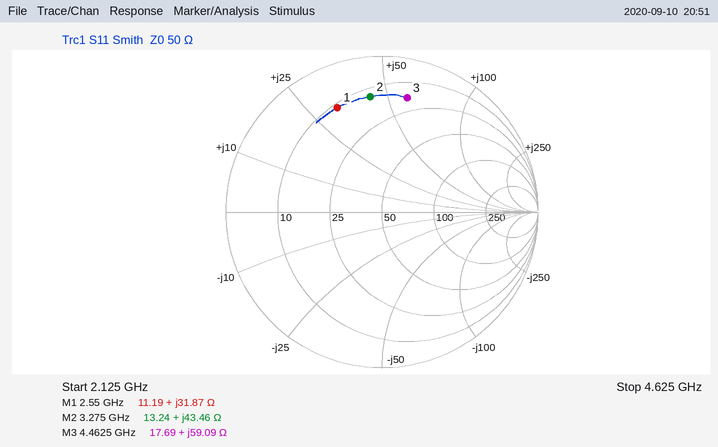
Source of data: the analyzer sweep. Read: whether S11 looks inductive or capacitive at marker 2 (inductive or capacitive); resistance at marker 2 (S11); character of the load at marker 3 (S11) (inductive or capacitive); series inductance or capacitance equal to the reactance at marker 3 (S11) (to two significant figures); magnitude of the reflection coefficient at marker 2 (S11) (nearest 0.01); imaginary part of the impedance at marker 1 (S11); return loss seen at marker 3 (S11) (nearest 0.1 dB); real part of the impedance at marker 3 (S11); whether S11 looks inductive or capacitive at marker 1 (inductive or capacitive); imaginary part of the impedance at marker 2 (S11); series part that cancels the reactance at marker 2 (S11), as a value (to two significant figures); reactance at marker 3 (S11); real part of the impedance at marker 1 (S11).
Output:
inductive
13.24 Ω
inductive
2.1 nH
0.74
+31.87 Ω
2.5 dB
17.69 Ω
inductive
+43.46 Ω
1.1 pF
+59.09 Ω
11.19 Ω
